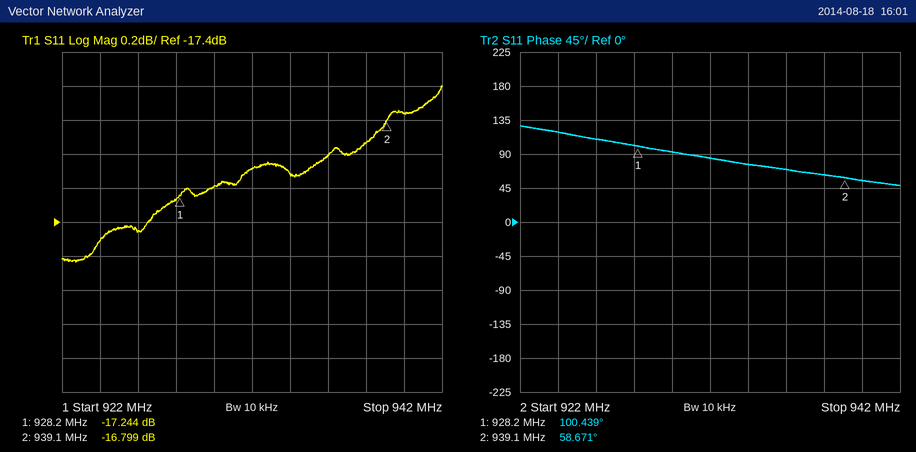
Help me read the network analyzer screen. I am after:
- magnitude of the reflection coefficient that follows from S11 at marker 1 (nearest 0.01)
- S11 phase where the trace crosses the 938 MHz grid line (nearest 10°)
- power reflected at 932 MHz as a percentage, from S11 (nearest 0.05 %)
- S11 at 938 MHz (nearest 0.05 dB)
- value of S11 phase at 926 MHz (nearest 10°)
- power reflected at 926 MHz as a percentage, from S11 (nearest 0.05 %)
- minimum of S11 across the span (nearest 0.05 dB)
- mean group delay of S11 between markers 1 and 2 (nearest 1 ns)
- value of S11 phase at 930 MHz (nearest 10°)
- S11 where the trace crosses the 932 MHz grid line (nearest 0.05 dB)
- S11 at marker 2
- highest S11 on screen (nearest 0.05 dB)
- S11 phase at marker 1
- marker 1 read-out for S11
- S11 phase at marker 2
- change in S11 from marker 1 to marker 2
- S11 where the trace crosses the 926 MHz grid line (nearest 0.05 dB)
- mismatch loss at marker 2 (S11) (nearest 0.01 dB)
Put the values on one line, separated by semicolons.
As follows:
0.14; 60°; 1.95 %; -16.95 dB; 110°; 1.80 %; -17.65 dB; 11 ns; 90°; -17.10 dB; -16.799 dB; -16.60 dB; 100.439°; -17.244 dB; 58.671°; 0.445 dB; -17.45 dB; 0.09 dB
